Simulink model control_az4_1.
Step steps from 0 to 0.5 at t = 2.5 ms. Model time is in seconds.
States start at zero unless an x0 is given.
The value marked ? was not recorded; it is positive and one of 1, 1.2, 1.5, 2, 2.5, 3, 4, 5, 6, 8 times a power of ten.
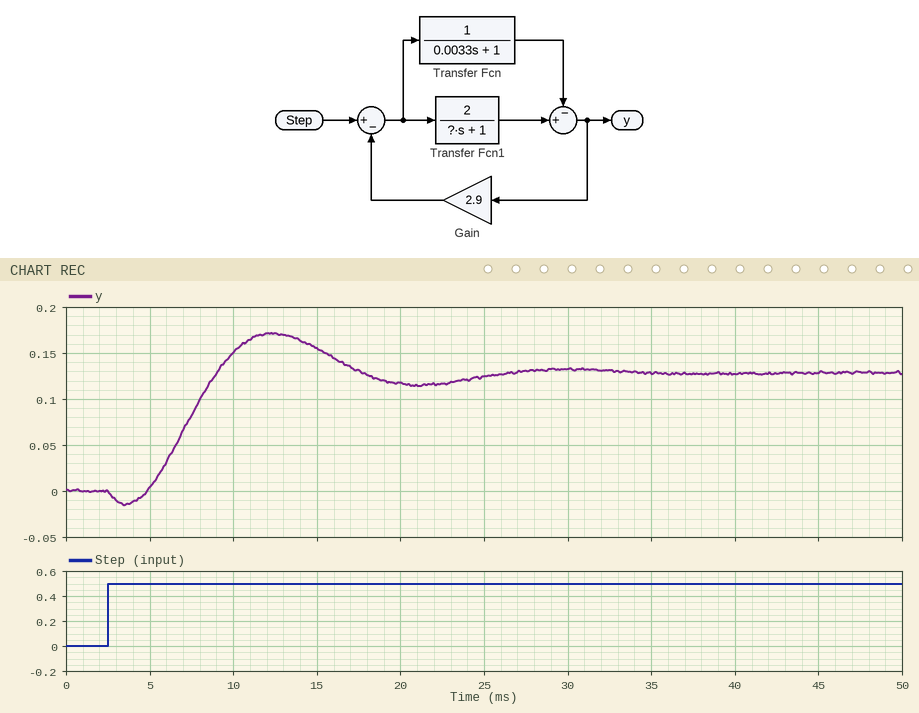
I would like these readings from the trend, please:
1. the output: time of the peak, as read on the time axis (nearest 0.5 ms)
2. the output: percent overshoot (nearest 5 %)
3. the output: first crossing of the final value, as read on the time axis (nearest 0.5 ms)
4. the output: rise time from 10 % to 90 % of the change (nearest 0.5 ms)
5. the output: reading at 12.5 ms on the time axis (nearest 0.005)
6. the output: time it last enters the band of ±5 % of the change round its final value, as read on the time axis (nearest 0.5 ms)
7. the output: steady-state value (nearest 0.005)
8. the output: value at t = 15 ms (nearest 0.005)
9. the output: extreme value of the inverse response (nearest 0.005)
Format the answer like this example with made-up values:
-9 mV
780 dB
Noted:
12.5 ms
35 %
9.0 ms
3.0 ms
0.170
24.5 ms
0.130
0.155
-0.015
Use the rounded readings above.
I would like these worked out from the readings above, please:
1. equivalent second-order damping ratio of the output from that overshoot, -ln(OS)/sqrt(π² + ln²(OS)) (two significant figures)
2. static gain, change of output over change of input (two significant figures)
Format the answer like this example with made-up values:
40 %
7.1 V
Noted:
0.32
0.26
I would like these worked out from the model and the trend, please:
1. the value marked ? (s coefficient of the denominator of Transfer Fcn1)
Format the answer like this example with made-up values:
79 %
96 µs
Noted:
0.008
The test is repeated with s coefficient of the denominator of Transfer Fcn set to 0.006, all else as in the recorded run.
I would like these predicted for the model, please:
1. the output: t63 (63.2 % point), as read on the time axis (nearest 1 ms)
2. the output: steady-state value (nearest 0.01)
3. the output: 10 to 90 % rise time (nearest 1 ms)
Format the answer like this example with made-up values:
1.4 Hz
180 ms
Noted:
5 ms
0.13
6 ms
